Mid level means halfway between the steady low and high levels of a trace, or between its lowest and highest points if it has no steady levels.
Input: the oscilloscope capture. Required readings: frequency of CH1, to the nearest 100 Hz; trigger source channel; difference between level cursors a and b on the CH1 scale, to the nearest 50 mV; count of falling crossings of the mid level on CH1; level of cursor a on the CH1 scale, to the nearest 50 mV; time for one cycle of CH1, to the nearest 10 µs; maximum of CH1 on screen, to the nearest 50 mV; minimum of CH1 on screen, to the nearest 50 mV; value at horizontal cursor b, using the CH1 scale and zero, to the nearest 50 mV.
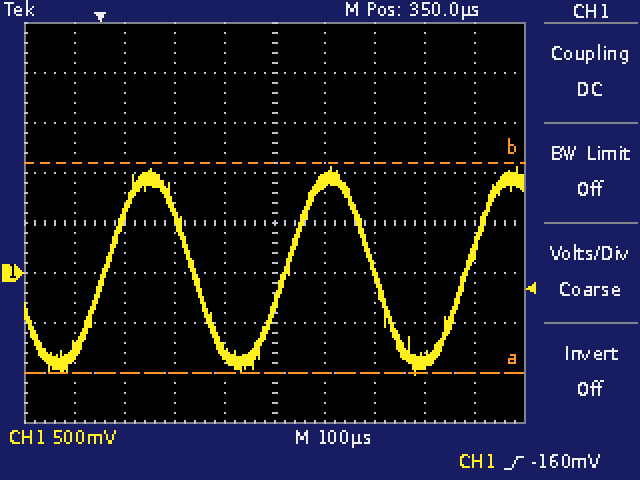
2.8 kHz
CH1
2.10 V
2
-1.00 V
360 µs
1.05 V
-1.00 V
1.10 V
